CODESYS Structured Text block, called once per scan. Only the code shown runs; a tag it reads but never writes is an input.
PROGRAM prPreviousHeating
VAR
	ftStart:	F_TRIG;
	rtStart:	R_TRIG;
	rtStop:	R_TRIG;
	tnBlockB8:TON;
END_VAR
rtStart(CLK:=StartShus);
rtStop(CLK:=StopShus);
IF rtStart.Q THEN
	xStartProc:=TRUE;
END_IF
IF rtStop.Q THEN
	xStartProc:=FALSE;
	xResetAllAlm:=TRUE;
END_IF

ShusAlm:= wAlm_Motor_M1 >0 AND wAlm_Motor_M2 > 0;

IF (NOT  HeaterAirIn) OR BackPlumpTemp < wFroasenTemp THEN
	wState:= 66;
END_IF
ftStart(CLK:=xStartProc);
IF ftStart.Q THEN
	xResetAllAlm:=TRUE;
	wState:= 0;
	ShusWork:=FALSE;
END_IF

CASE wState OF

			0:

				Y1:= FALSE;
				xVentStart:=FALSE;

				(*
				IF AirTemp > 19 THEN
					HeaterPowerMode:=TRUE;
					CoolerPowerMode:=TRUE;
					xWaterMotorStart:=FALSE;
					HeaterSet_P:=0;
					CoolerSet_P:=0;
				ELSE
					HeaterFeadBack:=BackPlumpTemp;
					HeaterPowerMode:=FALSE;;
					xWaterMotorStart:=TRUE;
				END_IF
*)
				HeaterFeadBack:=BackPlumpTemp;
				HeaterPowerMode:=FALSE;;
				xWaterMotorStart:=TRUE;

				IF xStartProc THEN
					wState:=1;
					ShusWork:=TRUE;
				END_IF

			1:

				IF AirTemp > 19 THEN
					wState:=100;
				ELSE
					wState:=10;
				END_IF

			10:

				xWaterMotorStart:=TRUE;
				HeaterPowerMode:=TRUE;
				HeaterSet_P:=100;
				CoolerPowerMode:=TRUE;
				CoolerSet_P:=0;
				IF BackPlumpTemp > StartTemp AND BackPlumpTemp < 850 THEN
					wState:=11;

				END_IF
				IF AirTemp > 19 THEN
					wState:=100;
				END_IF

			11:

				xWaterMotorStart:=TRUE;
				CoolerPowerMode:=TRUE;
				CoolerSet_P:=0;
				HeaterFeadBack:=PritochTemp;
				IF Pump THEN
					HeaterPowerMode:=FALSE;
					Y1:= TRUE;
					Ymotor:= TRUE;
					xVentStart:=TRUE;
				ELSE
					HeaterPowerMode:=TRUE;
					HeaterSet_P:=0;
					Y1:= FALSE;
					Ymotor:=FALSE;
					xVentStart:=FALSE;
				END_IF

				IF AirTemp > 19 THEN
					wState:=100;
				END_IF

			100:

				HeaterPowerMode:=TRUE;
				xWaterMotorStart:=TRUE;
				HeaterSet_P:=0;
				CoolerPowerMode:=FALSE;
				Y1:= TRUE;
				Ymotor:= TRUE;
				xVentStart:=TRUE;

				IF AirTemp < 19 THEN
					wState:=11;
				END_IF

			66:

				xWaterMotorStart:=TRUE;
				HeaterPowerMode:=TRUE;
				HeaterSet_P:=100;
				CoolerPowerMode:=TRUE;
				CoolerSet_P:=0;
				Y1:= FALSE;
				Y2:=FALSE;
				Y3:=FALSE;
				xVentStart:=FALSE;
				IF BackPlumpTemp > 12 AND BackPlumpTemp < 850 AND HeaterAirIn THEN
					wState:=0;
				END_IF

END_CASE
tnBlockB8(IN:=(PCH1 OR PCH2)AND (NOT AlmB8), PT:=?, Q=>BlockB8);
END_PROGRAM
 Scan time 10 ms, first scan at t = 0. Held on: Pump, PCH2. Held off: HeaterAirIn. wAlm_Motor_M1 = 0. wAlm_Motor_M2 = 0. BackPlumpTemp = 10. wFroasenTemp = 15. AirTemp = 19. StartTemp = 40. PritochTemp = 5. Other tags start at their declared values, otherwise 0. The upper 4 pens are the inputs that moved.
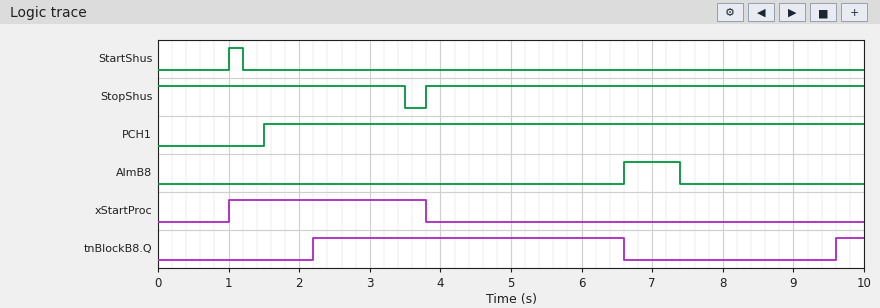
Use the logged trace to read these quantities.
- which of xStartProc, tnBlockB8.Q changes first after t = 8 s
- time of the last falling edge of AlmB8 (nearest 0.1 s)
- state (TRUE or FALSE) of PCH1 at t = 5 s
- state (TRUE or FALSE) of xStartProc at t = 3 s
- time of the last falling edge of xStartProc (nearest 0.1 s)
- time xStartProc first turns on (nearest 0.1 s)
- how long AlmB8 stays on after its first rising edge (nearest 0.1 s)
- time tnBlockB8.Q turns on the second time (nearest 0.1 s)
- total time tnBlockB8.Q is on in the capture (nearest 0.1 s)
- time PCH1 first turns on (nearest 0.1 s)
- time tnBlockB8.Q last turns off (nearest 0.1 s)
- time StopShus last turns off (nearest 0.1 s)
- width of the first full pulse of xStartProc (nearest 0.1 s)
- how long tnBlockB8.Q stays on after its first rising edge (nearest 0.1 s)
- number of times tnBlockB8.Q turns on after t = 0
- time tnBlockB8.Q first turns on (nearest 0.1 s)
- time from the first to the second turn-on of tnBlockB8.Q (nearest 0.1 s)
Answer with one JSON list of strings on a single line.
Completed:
["tnBlockB8.Q", "7.4 s", "TRUE", "TRUE", "3.8 s", "1.0 s", "0.8 s", "9.6 s", "4.8 s", "1.5 s", "6.6 s", "3.5 s", "2.8 s", "4.4 s", "2", "2.2 s", "7.4 s"]
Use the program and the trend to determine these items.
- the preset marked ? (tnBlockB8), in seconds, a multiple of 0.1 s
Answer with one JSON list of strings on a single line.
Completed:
["2.2 s"]
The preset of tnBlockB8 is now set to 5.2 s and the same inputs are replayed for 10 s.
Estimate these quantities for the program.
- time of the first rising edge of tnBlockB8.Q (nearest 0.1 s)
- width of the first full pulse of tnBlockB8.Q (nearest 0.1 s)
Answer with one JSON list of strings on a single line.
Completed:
["5.2 s", "1.4 s"]
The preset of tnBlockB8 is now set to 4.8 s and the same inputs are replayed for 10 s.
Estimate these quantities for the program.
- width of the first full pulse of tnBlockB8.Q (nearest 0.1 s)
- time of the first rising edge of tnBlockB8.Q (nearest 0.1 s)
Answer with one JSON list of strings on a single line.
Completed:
["1.8 s", "4.8 s"]
